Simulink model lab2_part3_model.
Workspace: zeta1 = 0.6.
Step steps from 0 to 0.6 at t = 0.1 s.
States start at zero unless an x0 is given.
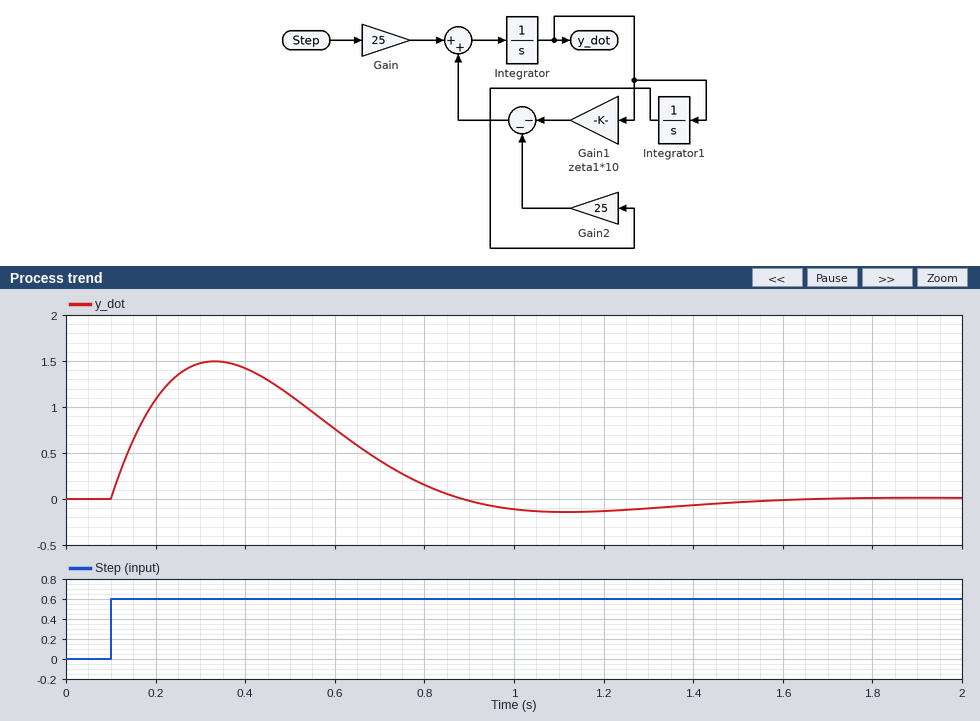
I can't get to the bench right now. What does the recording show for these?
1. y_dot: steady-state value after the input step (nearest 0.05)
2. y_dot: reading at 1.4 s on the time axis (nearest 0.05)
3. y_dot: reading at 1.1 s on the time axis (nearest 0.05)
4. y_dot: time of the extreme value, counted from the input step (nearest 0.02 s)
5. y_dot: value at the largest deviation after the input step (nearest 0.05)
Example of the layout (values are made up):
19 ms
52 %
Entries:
0.00
-0.05
-0.15
0.24 s
1.50
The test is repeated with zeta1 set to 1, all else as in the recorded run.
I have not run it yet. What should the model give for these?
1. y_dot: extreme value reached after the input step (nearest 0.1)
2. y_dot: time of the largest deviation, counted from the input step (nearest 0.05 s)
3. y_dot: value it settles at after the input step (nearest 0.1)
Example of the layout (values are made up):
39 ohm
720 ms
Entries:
1.1
0.20 s
0.0
